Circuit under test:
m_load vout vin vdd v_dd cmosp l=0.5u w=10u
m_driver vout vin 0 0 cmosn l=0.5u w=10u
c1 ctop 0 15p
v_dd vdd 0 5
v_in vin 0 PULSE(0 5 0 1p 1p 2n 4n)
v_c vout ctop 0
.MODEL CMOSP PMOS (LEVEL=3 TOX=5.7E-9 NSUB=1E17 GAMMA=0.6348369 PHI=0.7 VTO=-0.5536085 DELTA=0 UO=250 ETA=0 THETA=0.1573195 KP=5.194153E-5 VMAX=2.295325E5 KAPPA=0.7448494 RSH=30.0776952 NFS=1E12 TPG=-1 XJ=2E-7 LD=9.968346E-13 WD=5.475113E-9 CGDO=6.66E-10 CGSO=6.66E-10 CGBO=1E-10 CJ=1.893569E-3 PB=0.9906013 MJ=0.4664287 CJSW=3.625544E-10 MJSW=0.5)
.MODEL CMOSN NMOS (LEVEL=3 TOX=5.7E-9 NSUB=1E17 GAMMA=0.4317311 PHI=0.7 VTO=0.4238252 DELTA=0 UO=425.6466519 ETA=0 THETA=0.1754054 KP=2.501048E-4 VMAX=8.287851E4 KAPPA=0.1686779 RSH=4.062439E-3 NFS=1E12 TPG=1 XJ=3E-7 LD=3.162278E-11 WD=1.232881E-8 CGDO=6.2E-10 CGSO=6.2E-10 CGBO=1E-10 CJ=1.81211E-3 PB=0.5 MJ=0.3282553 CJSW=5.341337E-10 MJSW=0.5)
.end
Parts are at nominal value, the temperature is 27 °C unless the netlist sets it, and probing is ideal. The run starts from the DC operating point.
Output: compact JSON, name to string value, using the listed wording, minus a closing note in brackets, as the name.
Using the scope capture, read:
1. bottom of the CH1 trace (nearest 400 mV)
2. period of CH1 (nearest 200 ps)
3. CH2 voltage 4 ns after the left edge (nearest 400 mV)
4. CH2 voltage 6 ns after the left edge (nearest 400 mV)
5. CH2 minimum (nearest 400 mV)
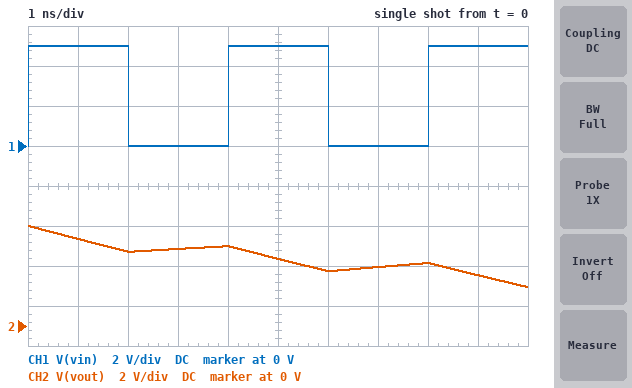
{"bottom of the CH1 trace": "0 V", "period of CH1": "4.0 ns", "CH2 voltage 4 ns after the left edge": "4.0 V", "CH2 voltage 6 ns after the left edge": "2.8 V", "CH2 minimum": "2.0 V"}
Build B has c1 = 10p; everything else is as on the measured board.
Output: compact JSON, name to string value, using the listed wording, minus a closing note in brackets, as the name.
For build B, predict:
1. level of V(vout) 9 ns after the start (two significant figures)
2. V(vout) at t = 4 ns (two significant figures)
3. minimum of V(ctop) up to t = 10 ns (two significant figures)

{"level of V(vout) 9 ns after the start": "1.6 V", "V(vout) at t = 4 ns": "3.6 V", "minimum of V(ctop) up to t = 10 ns": "840 mV"}
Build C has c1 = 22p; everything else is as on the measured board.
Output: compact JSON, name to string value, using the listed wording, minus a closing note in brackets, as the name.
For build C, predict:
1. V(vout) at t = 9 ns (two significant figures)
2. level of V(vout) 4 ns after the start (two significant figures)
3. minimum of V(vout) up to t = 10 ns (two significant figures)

{"V(vout) at t = 9 ns": "3.2 V", "level of V(vout) 4 ns after the start": "4.3 V", "minimum of V(vout) up to t = 10 ns": "2.8 V"}
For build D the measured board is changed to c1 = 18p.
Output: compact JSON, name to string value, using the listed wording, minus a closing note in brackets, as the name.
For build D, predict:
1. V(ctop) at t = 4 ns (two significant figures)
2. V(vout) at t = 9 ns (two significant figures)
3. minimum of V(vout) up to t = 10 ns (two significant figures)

{"V(ctop) at t = 4 ns": "4.1 V", "V(vout) at t = 9 ns": "2.9 V", "minimum of V(vout) up to t = 10 ns": "2.4 V"}
